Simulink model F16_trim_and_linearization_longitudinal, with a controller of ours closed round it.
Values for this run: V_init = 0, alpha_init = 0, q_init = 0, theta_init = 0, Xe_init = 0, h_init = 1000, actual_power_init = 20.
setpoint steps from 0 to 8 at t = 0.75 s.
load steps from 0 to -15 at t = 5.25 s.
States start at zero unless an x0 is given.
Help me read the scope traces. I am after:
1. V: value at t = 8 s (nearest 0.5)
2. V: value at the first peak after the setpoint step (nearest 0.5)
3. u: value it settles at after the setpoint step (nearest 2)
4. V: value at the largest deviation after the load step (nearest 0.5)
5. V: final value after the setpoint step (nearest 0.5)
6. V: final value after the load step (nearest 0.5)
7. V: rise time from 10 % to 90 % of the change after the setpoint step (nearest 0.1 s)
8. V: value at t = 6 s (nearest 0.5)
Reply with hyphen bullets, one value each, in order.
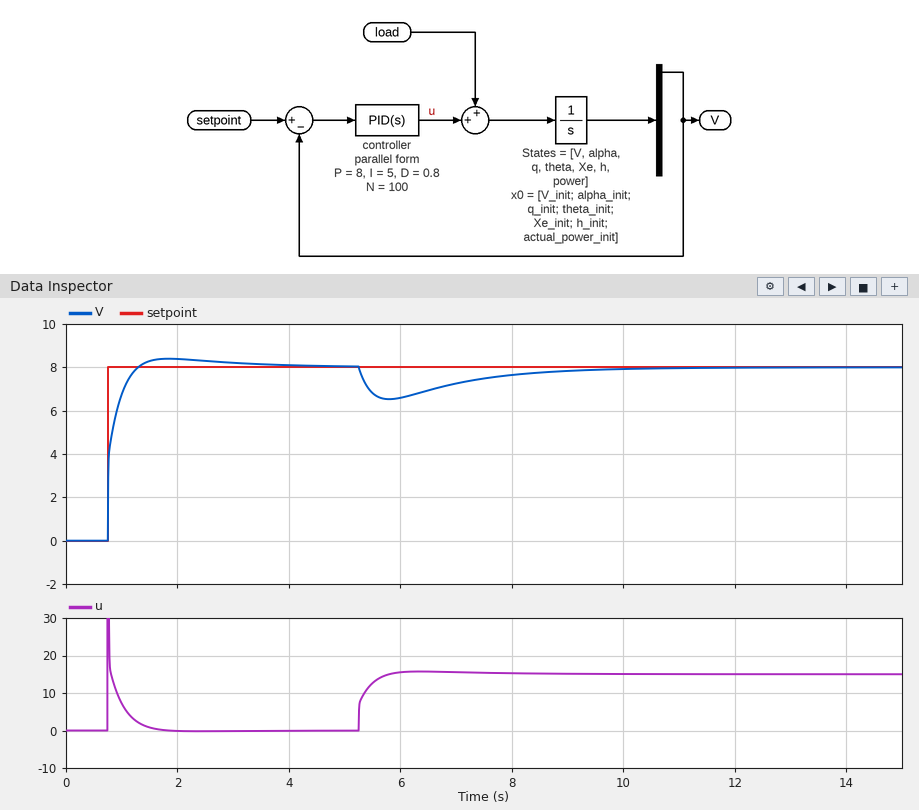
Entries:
- 7.5
- 8.5
- 0
- 6.5
- 8.0
- 8.0
- 0.3 s
- 6.5
